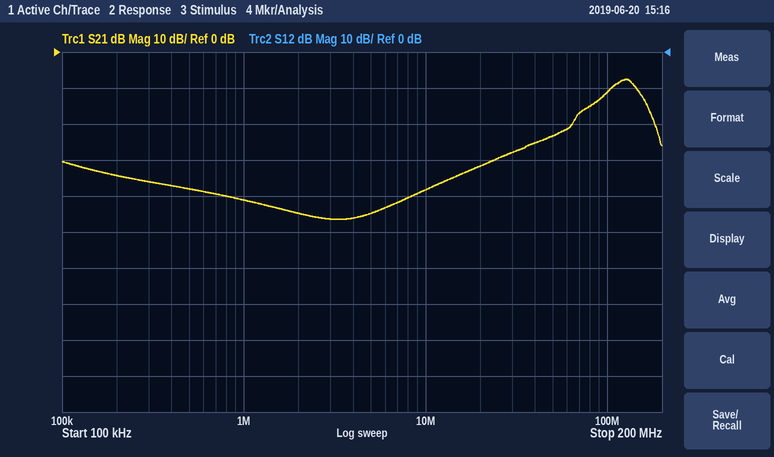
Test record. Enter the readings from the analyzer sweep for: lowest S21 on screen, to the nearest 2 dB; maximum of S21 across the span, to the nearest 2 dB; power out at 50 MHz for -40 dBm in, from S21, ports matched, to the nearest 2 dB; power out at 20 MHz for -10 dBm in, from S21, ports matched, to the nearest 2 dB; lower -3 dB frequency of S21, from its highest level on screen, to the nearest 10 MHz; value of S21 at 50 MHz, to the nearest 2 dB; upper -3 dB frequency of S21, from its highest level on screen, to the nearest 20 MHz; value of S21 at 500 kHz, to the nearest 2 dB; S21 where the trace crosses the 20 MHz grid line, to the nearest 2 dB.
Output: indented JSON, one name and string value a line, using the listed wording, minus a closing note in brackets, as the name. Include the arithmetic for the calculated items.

{
  "lowest S21 on screen, to the nearest 2 dB": "-46 dB",
  "maximum of S21 across the span, to the nearest 2 dB": "-8 dB",
  "power out at 50 MHz for -40 dBm in, from S21, ports matched, to the nearest 2 dB": "-40 dBm + (-24 dB) = -64 dBm",
  "power out at 20 MHz for -10 dBm in, from S21, ports matched, to the nearest 2 dB": "-10 dBm + (-32 dB) = -42 dBm",
  "lower -3 dB frequency of S21, from its highest level on screen, to the nearest 10 MHz": "100 MHz",
  "value of S21 at 50 MHz, to the nearest 2 dB": "-24 dB",
  "upper -3 dB frequency of S21, from its highest level on screen, to the nearest 20 MHz": "140 MHz",
  "value of S21 at 500 kHz, to the nearest 2 dB": "-38 dB",
  "S21 where the trace crosses the 20 MHz grid line, to the nearest 2 dB": "-32 dB"
}
